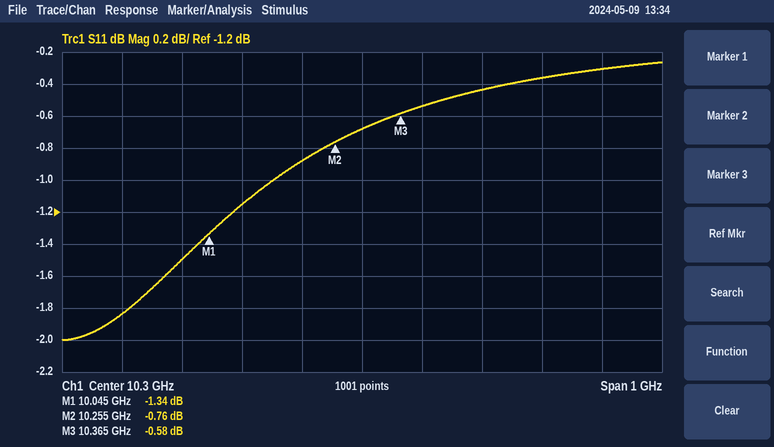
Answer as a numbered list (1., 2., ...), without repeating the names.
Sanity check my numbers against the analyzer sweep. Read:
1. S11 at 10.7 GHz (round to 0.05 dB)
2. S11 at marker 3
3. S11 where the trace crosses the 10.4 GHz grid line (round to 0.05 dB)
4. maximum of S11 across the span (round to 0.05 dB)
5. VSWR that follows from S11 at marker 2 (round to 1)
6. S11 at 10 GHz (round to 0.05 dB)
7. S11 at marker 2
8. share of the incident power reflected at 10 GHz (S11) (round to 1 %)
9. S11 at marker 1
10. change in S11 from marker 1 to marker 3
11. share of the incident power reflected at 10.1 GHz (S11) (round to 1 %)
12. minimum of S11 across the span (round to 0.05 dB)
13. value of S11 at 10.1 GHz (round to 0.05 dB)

1. -0.30 dB
2. -0.58 dB
3. -0.55 dB
4. -0.25 dB
5. 23
6. -1.50 dB
7. -0.76 dB
8. 71 %
9. -1.34 dB
10. 0.76 dB
11. 77 %
12. -2.00 dB
13. -1.15 dB
